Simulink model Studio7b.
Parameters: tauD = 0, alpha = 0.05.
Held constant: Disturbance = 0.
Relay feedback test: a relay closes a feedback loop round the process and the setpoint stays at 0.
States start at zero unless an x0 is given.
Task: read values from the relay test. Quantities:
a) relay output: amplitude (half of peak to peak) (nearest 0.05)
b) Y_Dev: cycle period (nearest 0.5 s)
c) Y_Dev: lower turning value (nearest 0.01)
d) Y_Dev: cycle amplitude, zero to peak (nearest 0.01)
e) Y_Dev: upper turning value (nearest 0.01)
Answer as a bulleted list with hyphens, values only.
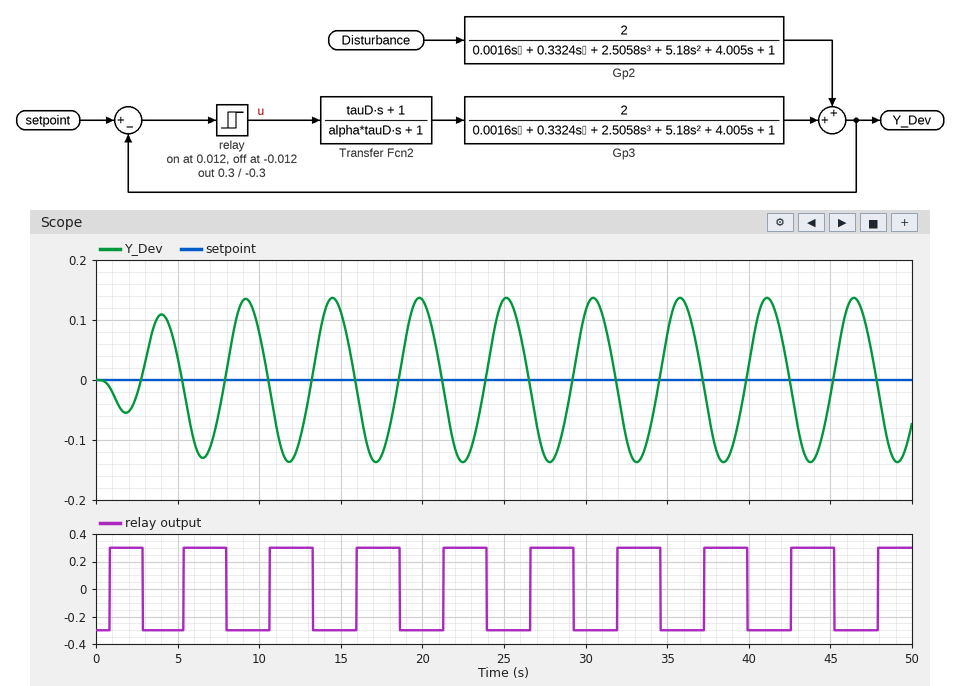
- 0.30
- 5.5 s
- -0.14
- 0.14
- 0.14
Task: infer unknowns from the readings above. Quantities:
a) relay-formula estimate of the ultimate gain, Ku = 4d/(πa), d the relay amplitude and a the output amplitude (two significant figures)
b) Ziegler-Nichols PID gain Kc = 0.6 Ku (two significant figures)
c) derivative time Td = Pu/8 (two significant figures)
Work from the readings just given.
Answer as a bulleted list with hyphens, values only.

- 2.7
- 1.6
- 0.69 s
